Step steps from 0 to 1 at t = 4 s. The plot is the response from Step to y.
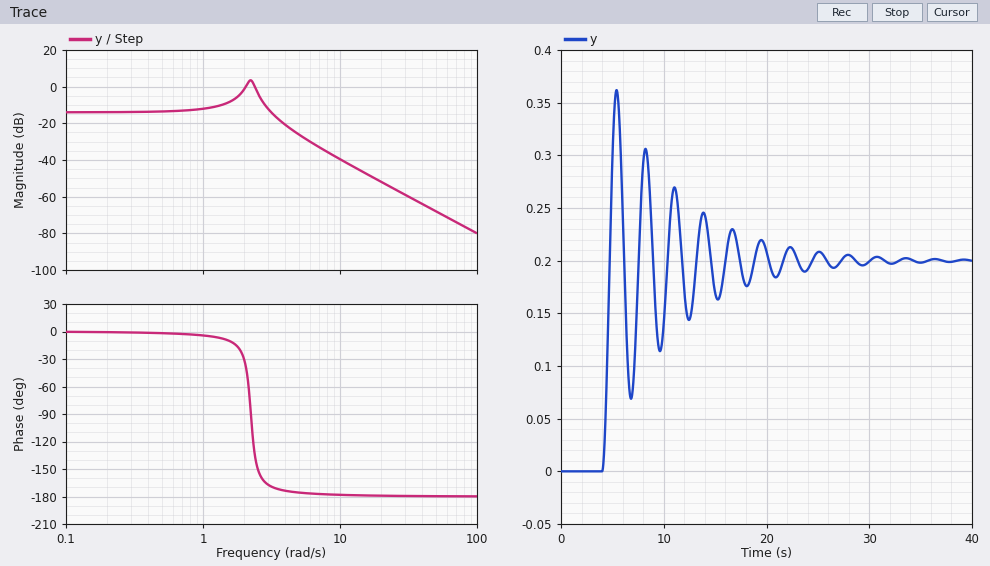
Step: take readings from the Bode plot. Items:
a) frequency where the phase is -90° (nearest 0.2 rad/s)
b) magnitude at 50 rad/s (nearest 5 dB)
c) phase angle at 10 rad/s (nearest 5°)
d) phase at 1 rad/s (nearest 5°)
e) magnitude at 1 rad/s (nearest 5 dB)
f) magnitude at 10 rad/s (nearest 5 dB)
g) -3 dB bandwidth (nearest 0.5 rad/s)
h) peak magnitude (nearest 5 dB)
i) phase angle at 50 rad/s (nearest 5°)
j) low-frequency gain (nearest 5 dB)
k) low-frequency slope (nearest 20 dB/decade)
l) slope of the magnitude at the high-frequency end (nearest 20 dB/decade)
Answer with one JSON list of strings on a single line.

["2.2 rad/s", "-70 dB", "-180°", "-5°", "-10 dB", "-40 dB", "3.5 rad/s", "5 dB", "-180°", "-15 dB", "0 dB/decade", "-40 dB/decade"]
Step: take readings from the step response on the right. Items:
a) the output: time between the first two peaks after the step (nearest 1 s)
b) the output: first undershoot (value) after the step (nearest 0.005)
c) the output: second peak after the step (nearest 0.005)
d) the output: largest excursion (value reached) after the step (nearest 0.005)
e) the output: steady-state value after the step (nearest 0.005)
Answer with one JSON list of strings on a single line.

["3 s", "0.070", "0.305", "0.360", "0.200"]
